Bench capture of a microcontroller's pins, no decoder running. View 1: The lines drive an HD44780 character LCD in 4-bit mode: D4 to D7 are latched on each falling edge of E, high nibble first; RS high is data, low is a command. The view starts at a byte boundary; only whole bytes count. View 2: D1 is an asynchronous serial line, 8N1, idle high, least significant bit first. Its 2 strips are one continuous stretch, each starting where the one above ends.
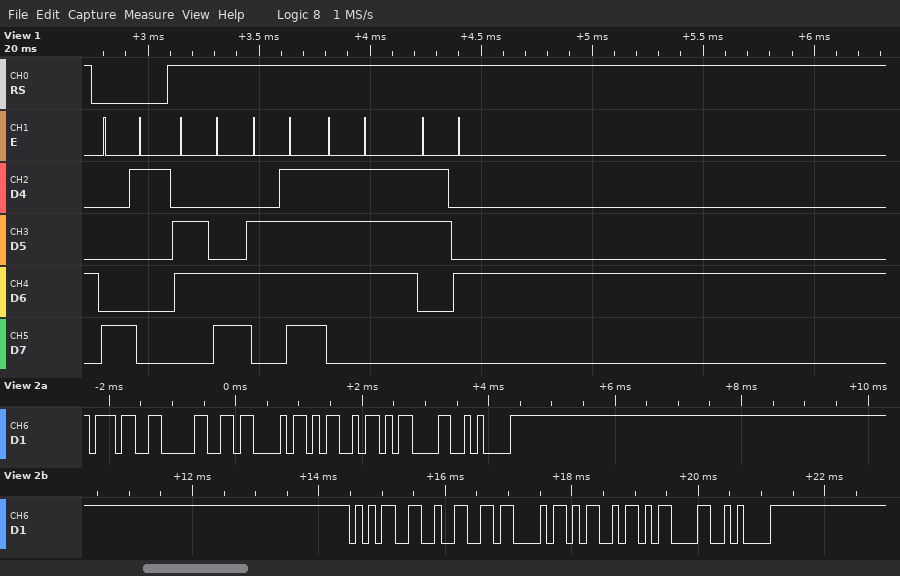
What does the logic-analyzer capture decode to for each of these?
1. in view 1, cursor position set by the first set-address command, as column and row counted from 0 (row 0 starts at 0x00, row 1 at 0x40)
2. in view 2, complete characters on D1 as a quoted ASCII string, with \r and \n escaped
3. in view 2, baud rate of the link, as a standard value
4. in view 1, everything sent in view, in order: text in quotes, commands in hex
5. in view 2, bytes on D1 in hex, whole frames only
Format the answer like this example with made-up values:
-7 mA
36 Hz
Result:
column 1, row 0
"70CM\r\n52CM\r\n"
9600 baud
0x81 "low4"
0x37 0x30 0x43 0x4D 0x0D 0x0A 0x35 0x32 0x43 0x4D 0x0D 0x0A
